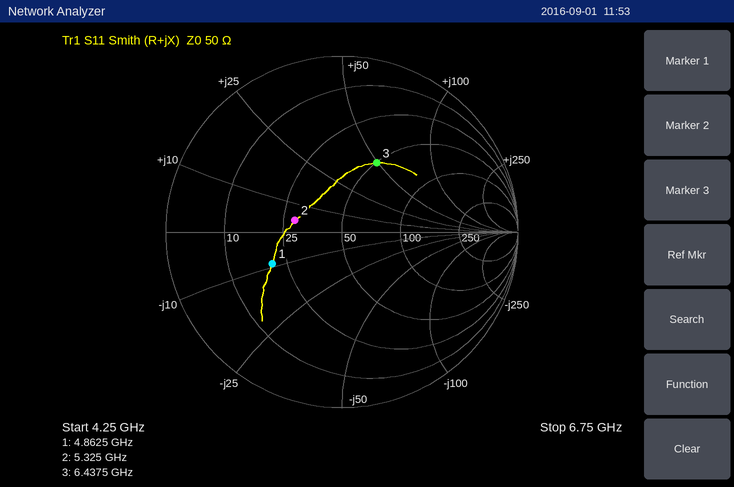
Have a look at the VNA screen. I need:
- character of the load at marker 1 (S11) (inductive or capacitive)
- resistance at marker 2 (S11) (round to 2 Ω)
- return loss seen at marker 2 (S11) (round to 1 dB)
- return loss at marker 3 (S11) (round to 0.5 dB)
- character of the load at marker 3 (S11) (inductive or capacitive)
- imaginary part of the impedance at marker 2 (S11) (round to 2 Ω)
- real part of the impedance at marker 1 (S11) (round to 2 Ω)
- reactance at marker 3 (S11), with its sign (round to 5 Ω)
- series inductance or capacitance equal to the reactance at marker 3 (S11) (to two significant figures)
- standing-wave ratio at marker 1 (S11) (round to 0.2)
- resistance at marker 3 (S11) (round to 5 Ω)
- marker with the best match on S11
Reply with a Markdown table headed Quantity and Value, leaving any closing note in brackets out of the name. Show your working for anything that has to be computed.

| Quantity | Value |
|---|---|
| character of the load at marker 1 (S11) | capacitive |
| resistance at marker 2 (S11) | 28 Ω |
| return loss seen at marker 2 (S11) | 11 dB |
| return loss at marker 3 (S11) | 7.0 dB |
| character of the load at marker 3 (S11) | inductive |
| imaginary part of the impedance at marker 2 (S11) | +4 Ω |
| real part of the impedance at marker 1 (S11) | 20 Ω |
| reactance at marker 3 (S11), with its sign | +50 Ω |
| series inductance or capacitance equal to the reactance at marker 3 (S11) | L = 50 Ω/(2π × 6.4375 GHz) ≈ 1.2 nH |
| standing-wave ratio at marker 1 (S11) | 2.6 |
| resistance at marker 3 (S11) | 50 Ω |
| marker with the best match on S11 | marker 2 |
